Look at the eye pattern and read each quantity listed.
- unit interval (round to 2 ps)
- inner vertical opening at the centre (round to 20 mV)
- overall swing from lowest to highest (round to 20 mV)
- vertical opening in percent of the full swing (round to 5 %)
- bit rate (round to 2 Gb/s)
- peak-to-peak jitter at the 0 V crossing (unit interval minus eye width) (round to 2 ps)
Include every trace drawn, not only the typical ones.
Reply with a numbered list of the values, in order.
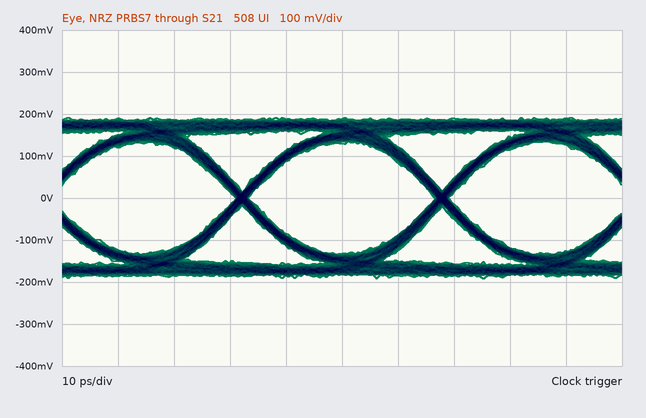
1. 36 ps
2. 260 mV
3. 380 mV
4. 70 %
5. 28 Gb/s
6. 2 ps
